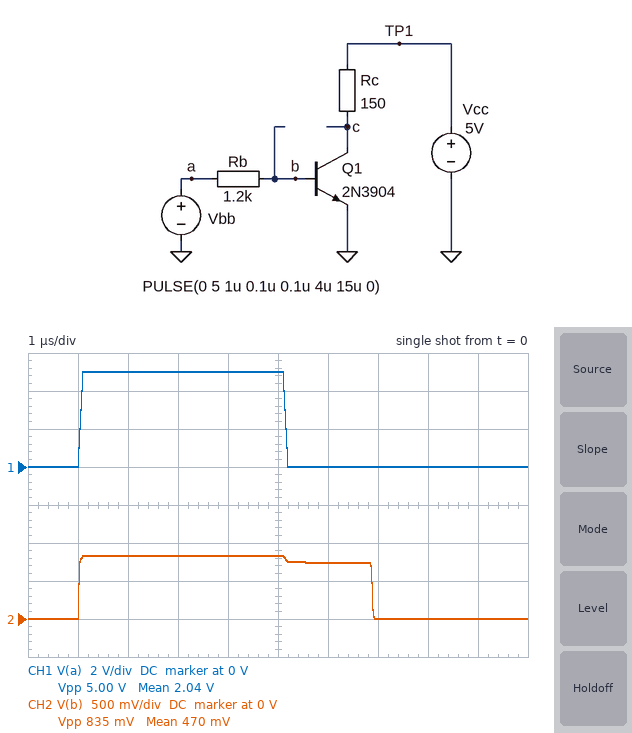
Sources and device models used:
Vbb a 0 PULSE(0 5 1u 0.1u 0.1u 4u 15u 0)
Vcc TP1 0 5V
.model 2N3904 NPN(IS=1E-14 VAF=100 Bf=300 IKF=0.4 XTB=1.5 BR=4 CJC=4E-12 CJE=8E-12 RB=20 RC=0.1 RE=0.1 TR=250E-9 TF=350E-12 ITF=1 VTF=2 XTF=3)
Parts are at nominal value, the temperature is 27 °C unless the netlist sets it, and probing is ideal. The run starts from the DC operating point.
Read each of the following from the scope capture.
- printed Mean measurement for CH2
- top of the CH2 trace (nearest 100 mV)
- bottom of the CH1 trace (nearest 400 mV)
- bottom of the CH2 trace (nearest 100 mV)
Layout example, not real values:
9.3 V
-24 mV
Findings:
470 mV
800 mV
0 V
0 V
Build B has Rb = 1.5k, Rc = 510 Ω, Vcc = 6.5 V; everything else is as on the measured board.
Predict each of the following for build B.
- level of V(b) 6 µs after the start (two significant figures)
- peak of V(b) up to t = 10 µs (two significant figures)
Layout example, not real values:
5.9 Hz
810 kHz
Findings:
720 mV
800 mV
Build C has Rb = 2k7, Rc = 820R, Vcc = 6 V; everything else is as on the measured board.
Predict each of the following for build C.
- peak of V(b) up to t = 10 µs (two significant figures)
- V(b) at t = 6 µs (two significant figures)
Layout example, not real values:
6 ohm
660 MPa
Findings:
760 mV
710 mV
